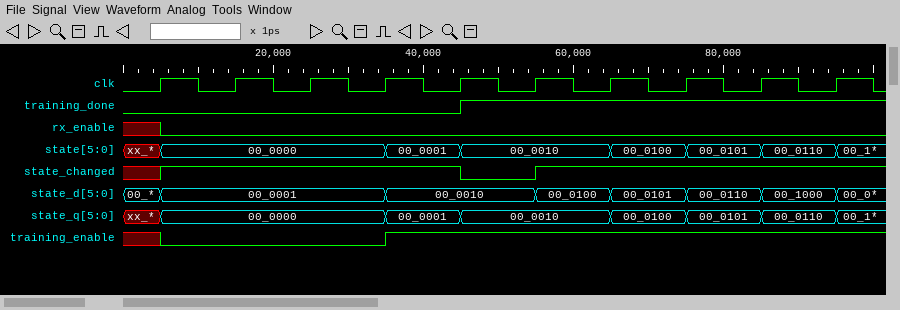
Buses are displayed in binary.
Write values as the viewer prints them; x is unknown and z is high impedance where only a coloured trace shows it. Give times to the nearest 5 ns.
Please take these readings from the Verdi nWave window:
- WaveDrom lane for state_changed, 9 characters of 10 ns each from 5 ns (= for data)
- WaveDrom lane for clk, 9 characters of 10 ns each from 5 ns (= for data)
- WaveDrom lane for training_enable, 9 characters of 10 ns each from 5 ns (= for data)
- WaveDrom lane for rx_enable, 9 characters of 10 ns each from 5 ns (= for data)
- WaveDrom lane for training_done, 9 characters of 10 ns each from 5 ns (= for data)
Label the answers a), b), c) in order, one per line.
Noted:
a) {name: 'state_changed', wave: '1...01...'}
b) {name: 'clk', wave: 'p........'}
c) {name: 'training_enable', wave: '0..1.....'}
d) {name: 'rx_enable', wave: '0........'}
e) {name: 'training_done', wave: '0...1....'}
